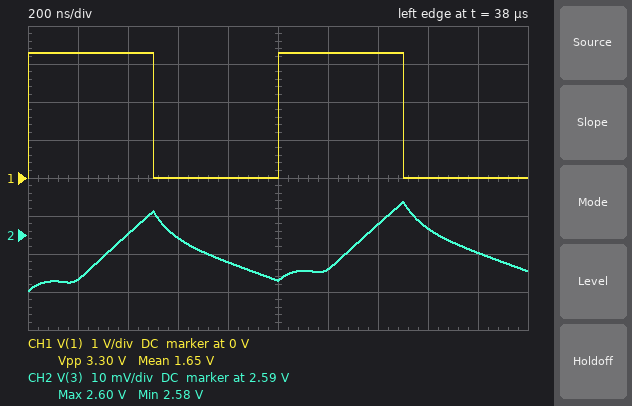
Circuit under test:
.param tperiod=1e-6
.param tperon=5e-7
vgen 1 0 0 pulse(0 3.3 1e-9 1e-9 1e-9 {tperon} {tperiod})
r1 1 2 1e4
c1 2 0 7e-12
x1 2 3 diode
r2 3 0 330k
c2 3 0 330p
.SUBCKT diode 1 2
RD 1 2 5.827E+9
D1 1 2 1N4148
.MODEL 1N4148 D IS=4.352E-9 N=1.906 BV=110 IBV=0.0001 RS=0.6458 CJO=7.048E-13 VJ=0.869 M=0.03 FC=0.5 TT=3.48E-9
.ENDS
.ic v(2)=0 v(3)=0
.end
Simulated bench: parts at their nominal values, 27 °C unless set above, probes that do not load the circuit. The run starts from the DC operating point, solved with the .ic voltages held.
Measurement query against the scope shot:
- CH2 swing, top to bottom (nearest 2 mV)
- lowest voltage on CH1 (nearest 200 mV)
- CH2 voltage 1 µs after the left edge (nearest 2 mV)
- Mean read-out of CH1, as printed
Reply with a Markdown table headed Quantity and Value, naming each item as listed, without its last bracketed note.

| Quantity | Value |
|---|---|
| CH2 swing, top to bottom | 24 mV |
| lowest voltage on CH1 | 0 V |
| CH2 voltage 1 µs after the left edge | 2.578 V |
| Mean read-out of CH1, as printed | 1.65 V |
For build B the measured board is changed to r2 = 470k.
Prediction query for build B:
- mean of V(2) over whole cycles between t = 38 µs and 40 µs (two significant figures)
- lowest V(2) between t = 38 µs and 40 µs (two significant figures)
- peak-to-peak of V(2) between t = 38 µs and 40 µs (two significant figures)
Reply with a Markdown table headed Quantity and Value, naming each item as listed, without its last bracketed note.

| Quantity | Value |
|---|---|
| mean of V(2) over whole cycles between t = 38 µs and 40 µs | 1.6 V |
| lowest V(2) between t = 38 µs and 40 µs | 4.6 mV |
| peak-to-peak of V(2) between t = 38 µs and 40 µs | 3.1 V |
